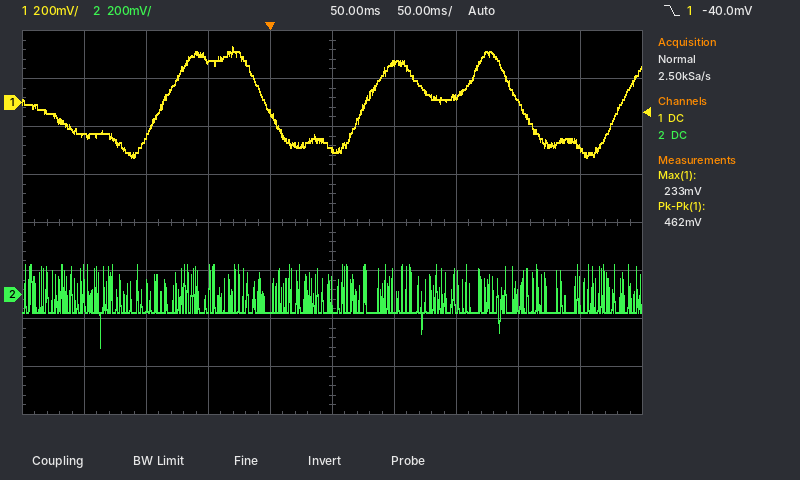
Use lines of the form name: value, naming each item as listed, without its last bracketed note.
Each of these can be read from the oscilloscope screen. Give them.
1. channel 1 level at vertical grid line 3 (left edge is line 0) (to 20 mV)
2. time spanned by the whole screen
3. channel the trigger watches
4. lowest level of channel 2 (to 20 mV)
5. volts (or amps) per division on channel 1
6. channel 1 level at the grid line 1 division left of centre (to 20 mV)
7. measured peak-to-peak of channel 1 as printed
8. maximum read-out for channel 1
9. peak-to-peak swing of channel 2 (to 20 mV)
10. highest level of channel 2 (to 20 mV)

channel 1 level at vertical grid line 3 (left edge is line 0): 180 mV
time spanned by the whole screen: 500 ms
channel the trigger watches: channel 1
lowest level of channel 2: -220 mV
volts (or amps) per division on channel 1: 200 mV
channel 1 level at the grid line 1 division left of centre: -40 mV
measured peak-to-peak of channel 1 as printed: 462 mV
maximum read-out for channel 1: 233 mV
peak-to-peak swing of channel 2: 340 mV
highest level of channel 2: 120 mV
